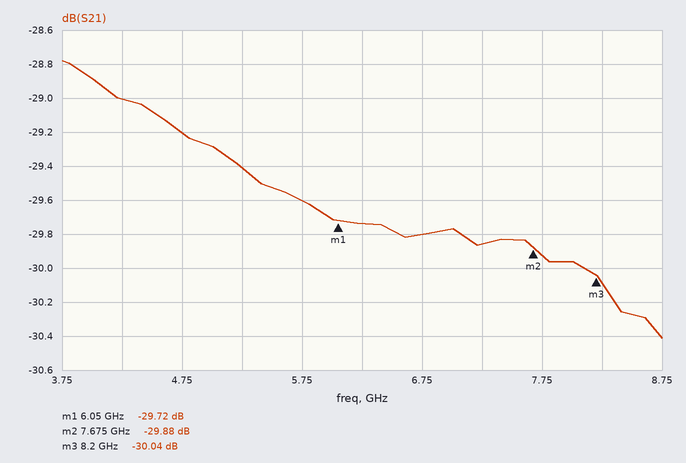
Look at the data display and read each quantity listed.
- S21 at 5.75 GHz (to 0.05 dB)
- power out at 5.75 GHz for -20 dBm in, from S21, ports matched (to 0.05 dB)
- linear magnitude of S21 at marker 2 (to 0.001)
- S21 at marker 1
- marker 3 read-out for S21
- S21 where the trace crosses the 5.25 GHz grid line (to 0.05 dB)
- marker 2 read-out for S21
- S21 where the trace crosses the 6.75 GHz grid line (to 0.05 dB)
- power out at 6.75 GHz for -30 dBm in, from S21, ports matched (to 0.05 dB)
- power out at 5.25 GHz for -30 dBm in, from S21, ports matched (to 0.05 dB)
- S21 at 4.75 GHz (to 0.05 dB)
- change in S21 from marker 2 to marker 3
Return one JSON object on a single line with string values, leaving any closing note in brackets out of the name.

{"S21 at 5.75 GHz": "-29.60 dB", "power out at 5.75 GHz for -20 dBm in, from S21, ports matched": "-49.60 dBm", "linear magnitude of S21 at marker 2": "0.032", "S21 at marker 1": "-29.72 dB", "marker 3 read-out for S21": "-30.04 dB", "S21 where the trace crosses the 5.25 GHz grid line": "-29.40 dB", "marker 2 read-out for S21": "-29.88 dB", "S21 where the trace crosses the 6.75 GHz grid line": "-29.80 dB", "power out at 6.75 GHz for -30 dBm in, from S21, ports matched": "-59.80 dBm", "power out at 5.25 GHz for -30 dBm in, from S21, ports matched": "-59.40 dBm", "S21 at 4.75 GHz": "-29.20 dB", "change in S21 from marker 2 to marker 3": "-0.16 dB"}
